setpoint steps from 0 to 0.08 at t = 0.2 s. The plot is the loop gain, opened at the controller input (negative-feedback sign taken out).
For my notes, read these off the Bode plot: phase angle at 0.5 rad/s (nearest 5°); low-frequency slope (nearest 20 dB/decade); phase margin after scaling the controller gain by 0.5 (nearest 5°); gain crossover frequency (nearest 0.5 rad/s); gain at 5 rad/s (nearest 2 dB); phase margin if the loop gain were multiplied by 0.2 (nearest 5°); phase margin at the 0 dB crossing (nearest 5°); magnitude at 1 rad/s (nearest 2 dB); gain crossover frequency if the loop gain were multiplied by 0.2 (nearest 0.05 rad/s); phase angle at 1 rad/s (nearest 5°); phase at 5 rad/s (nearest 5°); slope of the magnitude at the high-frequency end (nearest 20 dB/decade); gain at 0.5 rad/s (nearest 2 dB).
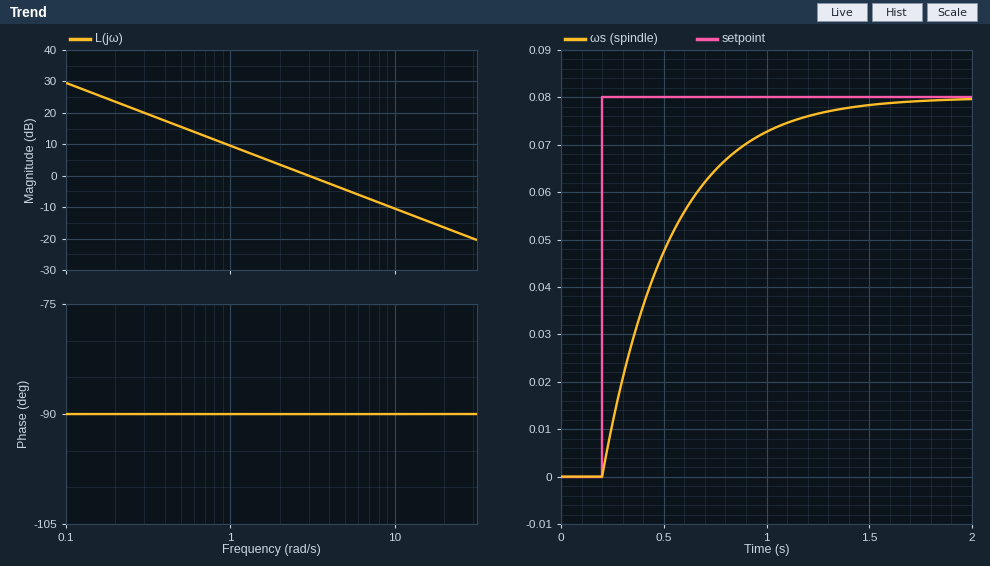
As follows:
-90°
-20 dB/decade
90°
3.0 rad/s
-4 dB
90°
90°
10 dB
0.60 rad/s
-90°
-90°
-20 dB/decade
16 dB
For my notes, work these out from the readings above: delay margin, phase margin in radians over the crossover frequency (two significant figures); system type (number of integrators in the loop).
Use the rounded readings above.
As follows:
0.52 s
1
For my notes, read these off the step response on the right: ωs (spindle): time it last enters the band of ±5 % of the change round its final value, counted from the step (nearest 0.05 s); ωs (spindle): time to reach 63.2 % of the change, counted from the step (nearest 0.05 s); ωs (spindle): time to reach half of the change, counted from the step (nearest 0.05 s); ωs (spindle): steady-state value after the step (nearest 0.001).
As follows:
1.00 s
0.35 s
0.25 s
0.080
